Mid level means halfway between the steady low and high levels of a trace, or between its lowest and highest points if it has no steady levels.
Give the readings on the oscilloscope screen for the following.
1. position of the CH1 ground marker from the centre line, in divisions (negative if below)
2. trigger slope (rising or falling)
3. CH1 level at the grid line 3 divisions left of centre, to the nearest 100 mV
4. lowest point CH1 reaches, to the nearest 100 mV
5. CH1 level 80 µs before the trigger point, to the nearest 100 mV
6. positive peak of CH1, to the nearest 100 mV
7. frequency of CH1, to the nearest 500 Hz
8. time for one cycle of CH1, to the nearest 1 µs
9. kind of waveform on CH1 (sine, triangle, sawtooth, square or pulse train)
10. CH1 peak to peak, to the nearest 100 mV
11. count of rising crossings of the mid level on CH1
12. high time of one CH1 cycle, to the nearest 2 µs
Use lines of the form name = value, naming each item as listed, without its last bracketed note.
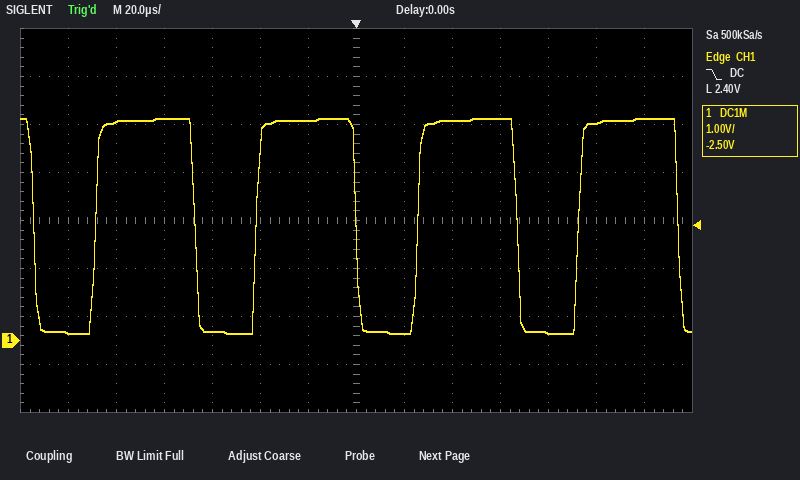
position of the CH1 ground marker from the centre line, in divisions = -2.5 div
trigger slope = falling
CH1 level at the grid line 3 divisions left of centre, to the nearest 100 mV = 200 mV
lowest point CH1 reaches, to the nearest 100 mV = 100 mV
CH1 level 80 µs before the trigger point, to the nearest 100 mV = 4.6 V
positive peak of CH1, to the nearest 100 mV = 4.6 V
frequency of CH1, to the nearest 500 Hz = 15.0 kHz
time for one cycle of CH1, to the nearest 1 µs = 67 µs
kind of waveform on CH1 = pulse train
CH1 peak to peak, to the nearest 100 mV = 4.5 V
count of rising crossings of the mid level on CH1 = 4
high time of one CH1 cycle, to the nearest 2 µs = 42 µs
